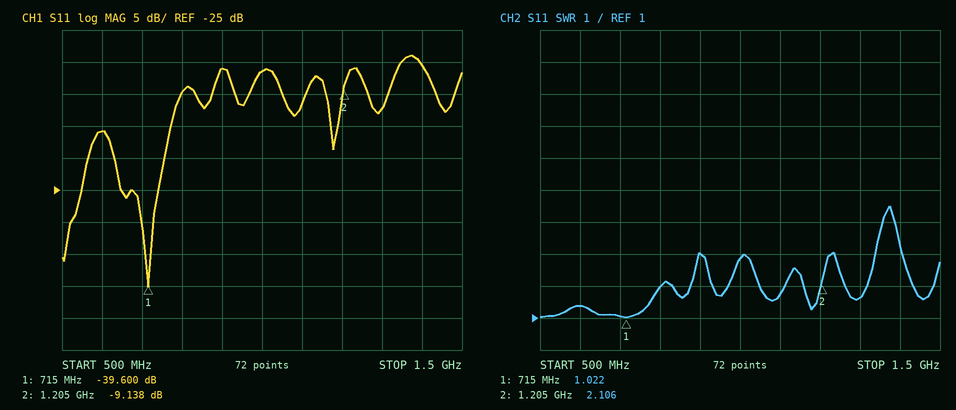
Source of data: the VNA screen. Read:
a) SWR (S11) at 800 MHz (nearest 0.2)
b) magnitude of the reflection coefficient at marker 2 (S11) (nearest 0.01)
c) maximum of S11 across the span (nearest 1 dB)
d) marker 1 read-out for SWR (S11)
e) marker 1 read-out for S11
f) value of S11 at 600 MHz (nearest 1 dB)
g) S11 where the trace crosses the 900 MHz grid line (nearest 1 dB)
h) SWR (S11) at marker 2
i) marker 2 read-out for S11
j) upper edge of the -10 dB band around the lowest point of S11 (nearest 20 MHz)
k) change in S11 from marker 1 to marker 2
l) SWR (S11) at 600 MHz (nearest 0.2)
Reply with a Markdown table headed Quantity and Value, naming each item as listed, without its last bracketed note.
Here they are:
| Quantity | Value |
|---|---|
| SWR (S11) at 800 MHz | 2.0 |
| magnitude of the reflection coefficient at marker 2 (S11) | 0.35 |
| maximum of S11 across the span | -4 dB |
| marker 1 read-out for SWR | 1.022 |
| marker 1 read-out for S11 | -39.600 dB |
| value of S11 at 600 MHz | -16 dB |
| S11 where the trace crosses the 900 MHz grid line | -6 dB |
| SWR (S11) at marker 2 | 2.106 |
| marker 2 read-out for S11 | -9.138 dB |
| upper edge of the -10 dB band around the lowest point of S11 | 800 MHz |
| change in S11 from marker 1 to marker 2 | 30.462 dB |
| SWR (S11) at 600 MHz | 1.4 |
